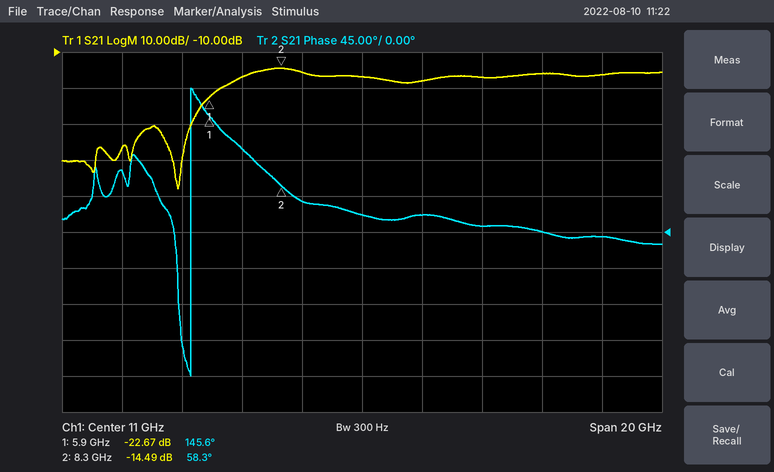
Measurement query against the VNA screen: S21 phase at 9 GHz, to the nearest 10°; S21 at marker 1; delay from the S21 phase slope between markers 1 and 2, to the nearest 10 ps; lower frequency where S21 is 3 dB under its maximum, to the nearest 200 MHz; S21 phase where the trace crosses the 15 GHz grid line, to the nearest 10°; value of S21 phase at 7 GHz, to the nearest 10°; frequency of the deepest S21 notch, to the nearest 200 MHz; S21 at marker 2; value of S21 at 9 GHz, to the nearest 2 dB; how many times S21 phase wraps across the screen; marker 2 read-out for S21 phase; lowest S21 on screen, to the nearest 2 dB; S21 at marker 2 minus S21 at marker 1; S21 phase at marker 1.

40°
-22.67 dB
100 ps
6.8 GHz
10°
100°
4.8 GHz
-14.49 dB
-16 dB
1
58.3°
-48 dB
8.18 dB
145.6°
